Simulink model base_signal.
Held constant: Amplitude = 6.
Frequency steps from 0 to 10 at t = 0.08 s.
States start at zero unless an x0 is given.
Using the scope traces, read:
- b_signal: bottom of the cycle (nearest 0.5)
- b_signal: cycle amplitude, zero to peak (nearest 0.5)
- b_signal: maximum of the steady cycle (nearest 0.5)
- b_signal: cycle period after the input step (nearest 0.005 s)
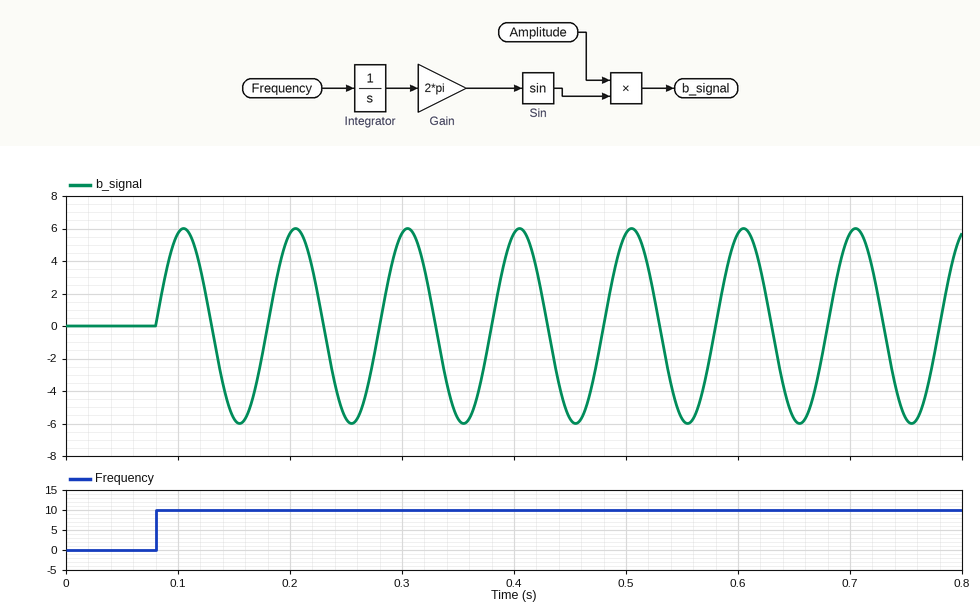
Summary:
-6.0
6.0
6.0
0.100 s
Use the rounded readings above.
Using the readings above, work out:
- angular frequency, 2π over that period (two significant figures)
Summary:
63 rad/s
